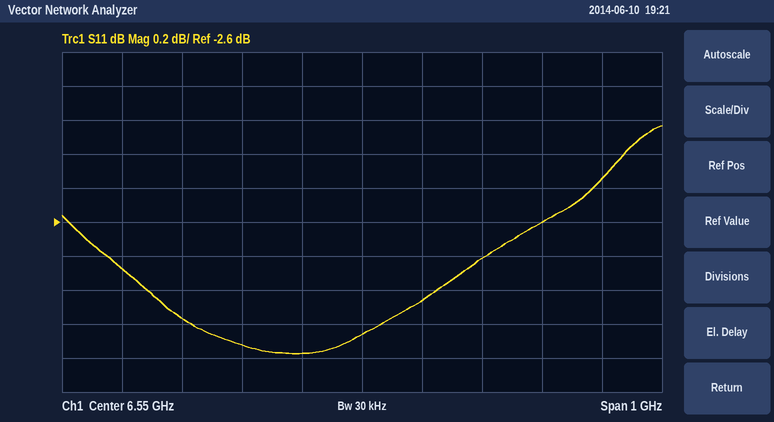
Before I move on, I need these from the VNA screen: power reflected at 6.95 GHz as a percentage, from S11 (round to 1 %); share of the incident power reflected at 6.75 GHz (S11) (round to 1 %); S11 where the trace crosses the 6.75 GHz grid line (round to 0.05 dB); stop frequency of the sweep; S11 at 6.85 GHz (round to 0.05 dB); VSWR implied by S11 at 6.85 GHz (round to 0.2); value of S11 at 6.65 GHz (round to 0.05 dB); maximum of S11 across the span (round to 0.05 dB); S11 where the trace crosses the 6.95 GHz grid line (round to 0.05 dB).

58 %
52 %
-2.80 dB
7.05 GHz
-2.60 dB
6.8
-3.05 dB
-2.05 dB
-2.35 dB
